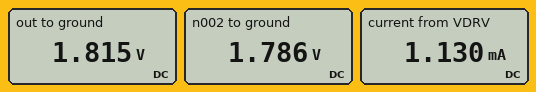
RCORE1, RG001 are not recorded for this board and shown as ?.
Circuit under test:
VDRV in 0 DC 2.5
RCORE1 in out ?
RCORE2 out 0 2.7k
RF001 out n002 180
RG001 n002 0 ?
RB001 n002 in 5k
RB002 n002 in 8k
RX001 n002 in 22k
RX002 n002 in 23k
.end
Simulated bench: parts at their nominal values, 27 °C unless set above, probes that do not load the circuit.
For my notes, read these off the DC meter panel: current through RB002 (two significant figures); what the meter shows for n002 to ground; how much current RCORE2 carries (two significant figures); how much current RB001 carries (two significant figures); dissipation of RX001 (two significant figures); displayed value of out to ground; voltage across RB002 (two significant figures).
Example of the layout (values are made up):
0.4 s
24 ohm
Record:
89 µA
1.786 V
670 µA
140 µA
23 µW
1.815 V
710 mV
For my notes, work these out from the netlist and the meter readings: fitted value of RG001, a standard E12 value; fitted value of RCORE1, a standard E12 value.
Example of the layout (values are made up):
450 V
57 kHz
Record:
3.9 kΩ
820 Ω
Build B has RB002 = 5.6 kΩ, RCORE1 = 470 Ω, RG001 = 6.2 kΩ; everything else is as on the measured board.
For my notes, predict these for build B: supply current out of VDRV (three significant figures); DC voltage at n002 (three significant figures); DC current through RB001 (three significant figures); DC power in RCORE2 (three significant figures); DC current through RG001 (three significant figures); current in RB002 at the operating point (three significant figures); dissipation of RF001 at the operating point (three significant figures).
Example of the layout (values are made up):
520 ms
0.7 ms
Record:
1.10 mA
2.06 V
88.6 µA
1.60 mW
332 µA
79.1 µA
2.80 µW
